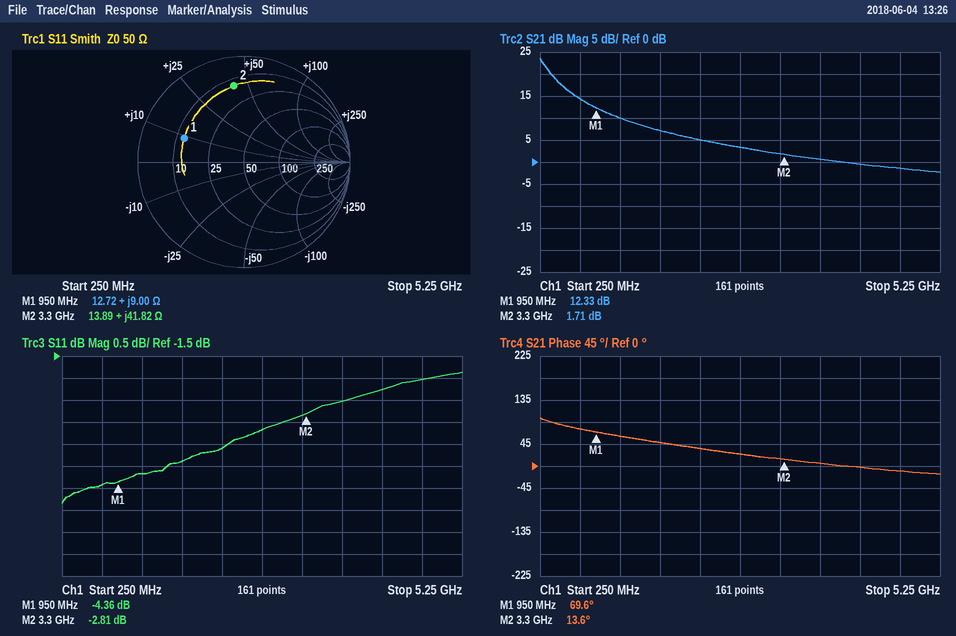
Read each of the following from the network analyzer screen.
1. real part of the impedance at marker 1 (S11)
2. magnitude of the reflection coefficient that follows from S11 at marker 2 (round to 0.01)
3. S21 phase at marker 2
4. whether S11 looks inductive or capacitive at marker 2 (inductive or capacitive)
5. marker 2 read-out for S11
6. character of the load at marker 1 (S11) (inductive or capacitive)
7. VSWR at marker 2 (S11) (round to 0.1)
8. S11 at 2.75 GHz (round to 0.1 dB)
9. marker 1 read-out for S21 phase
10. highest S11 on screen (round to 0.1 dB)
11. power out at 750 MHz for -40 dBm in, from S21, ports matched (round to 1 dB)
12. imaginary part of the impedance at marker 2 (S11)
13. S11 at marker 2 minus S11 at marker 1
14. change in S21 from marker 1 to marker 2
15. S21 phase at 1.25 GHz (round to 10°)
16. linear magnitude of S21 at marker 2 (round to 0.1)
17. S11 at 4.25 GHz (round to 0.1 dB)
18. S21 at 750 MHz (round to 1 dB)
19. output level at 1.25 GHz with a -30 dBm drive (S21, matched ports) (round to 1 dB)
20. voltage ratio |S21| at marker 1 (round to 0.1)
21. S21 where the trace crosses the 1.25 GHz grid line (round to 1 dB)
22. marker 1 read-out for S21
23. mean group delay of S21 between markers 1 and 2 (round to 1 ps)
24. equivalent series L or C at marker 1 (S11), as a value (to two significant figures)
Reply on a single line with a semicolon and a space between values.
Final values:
12.72 Ω; 0.72; 13.6°; inductive; -2.81 dB; inductive; 6.2; -3.2 dB; 69.6°; -1.9 dB; -26 dBm; +41.82 Ω; 1.55 dB; -10.62 dB; 60°; 1.2; -2.3 dB; 14 dB; -20 dBm; 4.1; 10 dB; 12.33 dB; 66 ps; 1.5 nH
